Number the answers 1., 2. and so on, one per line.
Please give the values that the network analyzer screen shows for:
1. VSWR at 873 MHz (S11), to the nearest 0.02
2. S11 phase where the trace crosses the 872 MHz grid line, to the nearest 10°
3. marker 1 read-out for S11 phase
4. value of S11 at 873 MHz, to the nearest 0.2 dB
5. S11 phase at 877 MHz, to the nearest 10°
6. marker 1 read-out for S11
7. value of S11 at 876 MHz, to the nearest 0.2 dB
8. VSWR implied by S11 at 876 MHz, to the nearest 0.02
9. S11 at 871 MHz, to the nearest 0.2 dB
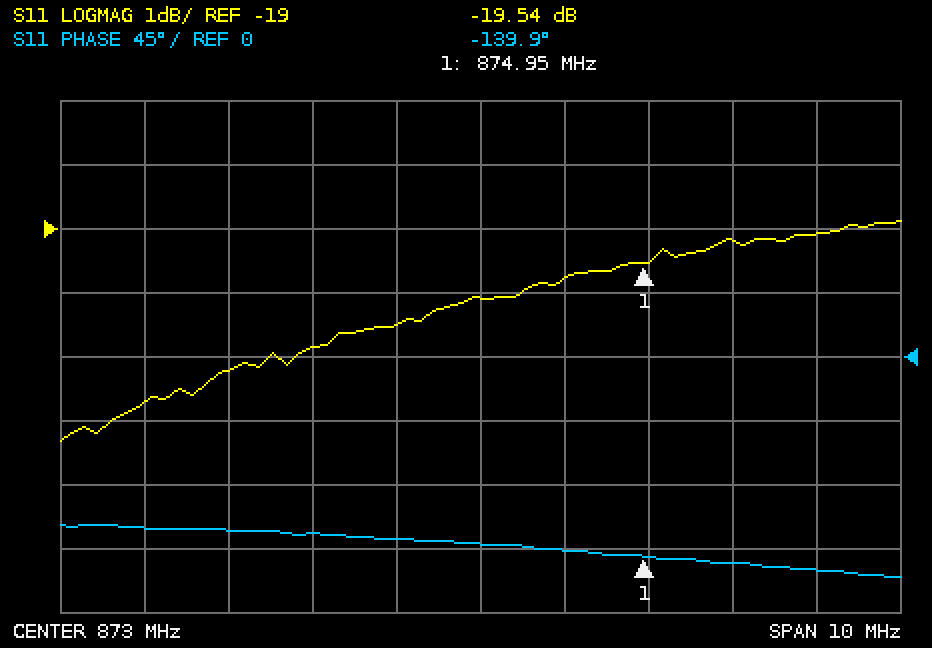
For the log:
1. 1.22
2. -130°
3. -139.9°
4. -20.0 dB
5. -150°
6. -19.54 dB
7. -19.2 dB
8. 1.24
9. -20.8 dB
